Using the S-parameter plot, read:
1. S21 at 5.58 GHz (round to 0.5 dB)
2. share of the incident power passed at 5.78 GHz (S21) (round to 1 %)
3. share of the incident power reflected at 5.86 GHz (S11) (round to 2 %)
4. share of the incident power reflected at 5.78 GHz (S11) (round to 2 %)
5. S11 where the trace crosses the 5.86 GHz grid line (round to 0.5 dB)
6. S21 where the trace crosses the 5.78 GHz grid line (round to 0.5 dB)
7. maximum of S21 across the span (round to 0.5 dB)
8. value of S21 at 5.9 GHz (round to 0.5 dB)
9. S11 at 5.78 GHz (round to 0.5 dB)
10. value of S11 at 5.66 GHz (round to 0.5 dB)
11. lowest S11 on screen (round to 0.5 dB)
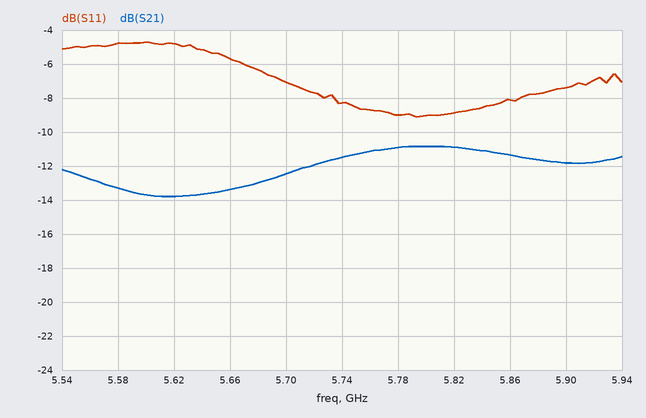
-13.5 dB
8 %
16 %
12 %
-8.0 dB
-11.0 dB
-11.0 dB
-12.0 dB
-9.0 dB
-5.5 dB
-9.0 dB
